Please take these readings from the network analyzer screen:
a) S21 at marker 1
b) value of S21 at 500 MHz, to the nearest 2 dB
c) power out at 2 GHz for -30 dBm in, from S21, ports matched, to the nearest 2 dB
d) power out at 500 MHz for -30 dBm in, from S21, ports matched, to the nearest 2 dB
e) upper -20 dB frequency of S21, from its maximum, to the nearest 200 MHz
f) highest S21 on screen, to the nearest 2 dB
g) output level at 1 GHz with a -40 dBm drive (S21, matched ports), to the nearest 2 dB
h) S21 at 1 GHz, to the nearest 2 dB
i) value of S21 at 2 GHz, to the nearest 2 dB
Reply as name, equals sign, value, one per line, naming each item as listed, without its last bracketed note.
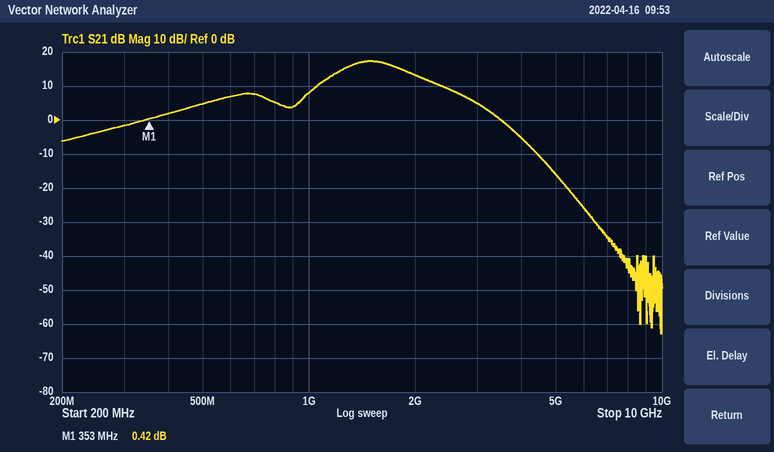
S21 at marker 1 = 0.42 dB
value of S21 at 500 MHz, to the nearest 2 dB = 4 dB
power out at 2 GHz for -30 dBm in, from S21, ports matched, to the nearest 2 dB = -16 dBm
power out at 500 MHz for -30 dBm in, from S21, ports matched, to the nearest 2 dB = -26 dBm
upper -20 dB frequency of S21, from its maximum, to the nearest 200 MHz = 3.8 GHz
highest S21 on screen, to the nearest 2 dB = 18 dB
output level at 1 GHz with a -40 dBm drive (S21, matched ports), to the nearest 2 dB = -32 dBm
S21 at 1 GHz, to the nearest 2 dB = 8 dB
value of S21 at 2 GHz, to the nearest 2 dB = 14 dB
